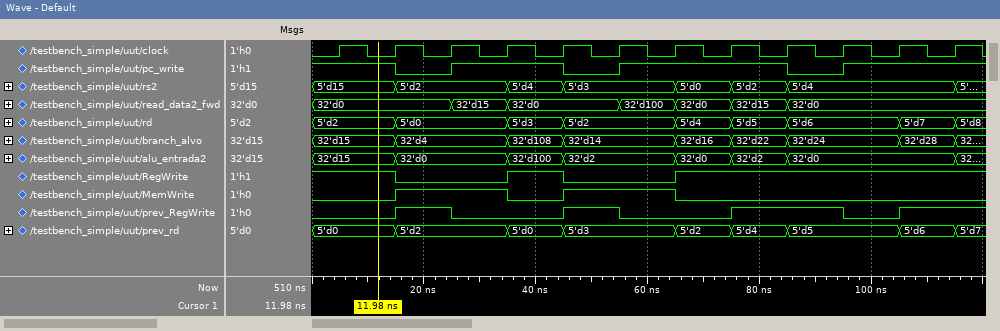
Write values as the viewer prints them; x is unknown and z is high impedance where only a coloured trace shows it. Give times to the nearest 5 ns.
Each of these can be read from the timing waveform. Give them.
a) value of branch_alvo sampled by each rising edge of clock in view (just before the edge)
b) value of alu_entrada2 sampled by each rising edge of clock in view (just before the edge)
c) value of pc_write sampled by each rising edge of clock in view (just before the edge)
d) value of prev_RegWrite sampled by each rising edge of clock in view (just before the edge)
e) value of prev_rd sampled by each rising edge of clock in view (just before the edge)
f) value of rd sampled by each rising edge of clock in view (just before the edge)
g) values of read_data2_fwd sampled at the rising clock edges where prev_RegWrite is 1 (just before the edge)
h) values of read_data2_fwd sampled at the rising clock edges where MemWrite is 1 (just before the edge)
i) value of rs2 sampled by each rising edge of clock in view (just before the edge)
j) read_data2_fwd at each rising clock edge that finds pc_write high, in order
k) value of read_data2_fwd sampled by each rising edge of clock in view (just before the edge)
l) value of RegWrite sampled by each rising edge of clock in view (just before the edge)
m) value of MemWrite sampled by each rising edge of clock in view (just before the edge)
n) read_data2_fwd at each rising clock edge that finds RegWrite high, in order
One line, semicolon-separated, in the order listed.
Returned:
32'd15, 32'd15, 32'd4, 32'd4, 32'd108, 32'd14, 32'd14, 32'd16, 32'd22, 32'd24, 32'd24, 32'd28; 32'd15, 32'd15, 32'd0, 32'd0, 32'd100, 32'd2, 32'd2, 32'd0, 32'd2, 32'd0, 32'd0, 32'd0; 1 1 0 1 1 0 1 1 1 0 1 1; 0 0 1 0 0 1 0 0 1 1 0 1; 5'd0, 5'd0, 5'd2, 5'd2, 5'd0, 5'd3, 5'd3, 5'd2, 5'd4, 5'd5, 5'd5, 5'd6; 5'd2, 5'd2, 5'd0, 5'd0, 5'd3, 5'd2, 5'd2, 5'd4, 5'd5, 5'd6, 5'd6, 5'd7; 32'd0, 32'd0, 32'd15, 32'd0, 32'd0; 32'd0, 32'd15, 32'd0, 32'd100; 5'd15, 5'd15, 5'd2, 5'd2, 5'd4, 5'd3, 5'd3, 5'd0, 5'd2, 5'd4, 5'd4, 5'd4; 32'd0, 32'd0, 32'd15, 32'd0, 32'd100, 32'd0, 32'd15, 32'd0, 32'd0; 32'd0, 32'd0, 32'd0, 32'd15, 32'd0, 32'd0, 32'd100, 32'd0, 32'd15, 32'd0, 32'd0, 32'd0; 1 1 0 0 1 0 0 1 1 1 1 1; 0 0 1 1 0 1 1 0 0 0 0 0; 32'd0, 32'd0, 32'd0, 32'd0, 32'd15, 32'd0, 32'd0, 32'd0
